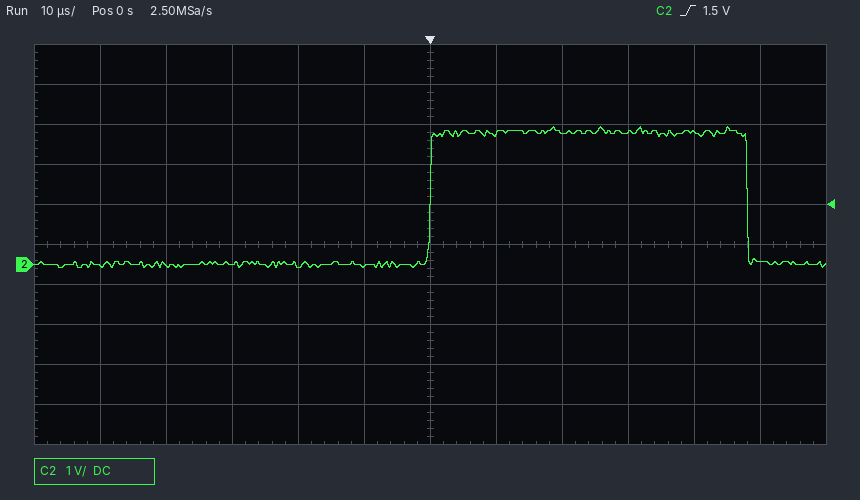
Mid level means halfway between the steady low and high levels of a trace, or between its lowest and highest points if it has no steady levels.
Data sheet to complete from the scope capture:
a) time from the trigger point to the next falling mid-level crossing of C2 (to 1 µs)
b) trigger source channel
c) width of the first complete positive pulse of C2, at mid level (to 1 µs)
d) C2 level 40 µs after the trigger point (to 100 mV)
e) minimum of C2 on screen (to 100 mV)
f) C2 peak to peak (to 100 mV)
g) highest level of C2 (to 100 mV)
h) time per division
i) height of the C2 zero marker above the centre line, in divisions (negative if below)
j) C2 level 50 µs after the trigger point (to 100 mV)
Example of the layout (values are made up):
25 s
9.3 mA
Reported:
48 µs
C2
48 µs
3.3 V
-100 mV
3.5 V
3.4 V
10 µs
-0.5 div
100 mV
